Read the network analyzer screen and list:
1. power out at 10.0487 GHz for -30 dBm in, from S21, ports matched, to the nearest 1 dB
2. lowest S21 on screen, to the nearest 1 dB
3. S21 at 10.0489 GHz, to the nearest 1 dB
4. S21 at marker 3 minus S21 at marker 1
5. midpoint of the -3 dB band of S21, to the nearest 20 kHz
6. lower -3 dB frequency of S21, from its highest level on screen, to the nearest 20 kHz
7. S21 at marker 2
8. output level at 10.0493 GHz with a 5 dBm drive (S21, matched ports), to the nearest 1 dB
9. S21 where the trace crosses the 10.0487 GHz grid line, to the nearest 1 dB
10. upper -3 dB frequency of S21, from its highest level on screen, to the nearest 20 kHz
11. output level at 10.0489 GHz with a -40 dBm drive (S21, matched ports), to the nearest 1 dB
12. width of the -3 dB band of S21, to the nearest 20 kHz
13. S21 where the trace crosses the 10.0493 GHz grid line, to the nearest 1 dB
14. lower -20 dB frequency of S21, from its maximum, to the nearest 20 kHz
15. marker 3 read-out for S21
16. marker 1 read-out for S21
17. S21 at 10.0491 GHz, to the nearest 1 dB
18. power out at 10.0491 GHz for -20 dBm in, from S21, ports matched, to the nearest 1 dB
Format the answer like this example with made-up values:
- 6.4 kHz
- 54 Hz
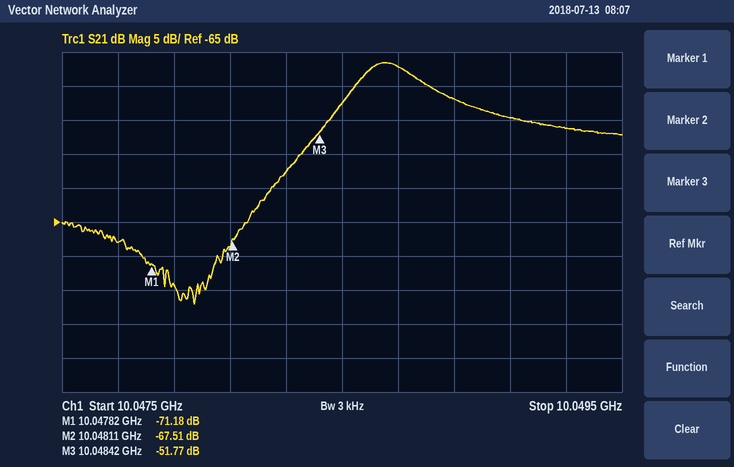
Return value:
- -72 dBm
- -77 dB
- -47 dB
- 19.41 dB
- 10.04868 GHz
- 10.04856 GHz
- -67.51 dB
- -46 dBm
- -42 dB
- 10.04880 GHz
- -87 dBm
- 240 kHz
- -51 dB
- 10.04822 GHz
- -51.77 dB
- -71.18 dB
- -50 dB
- -70 dBm
